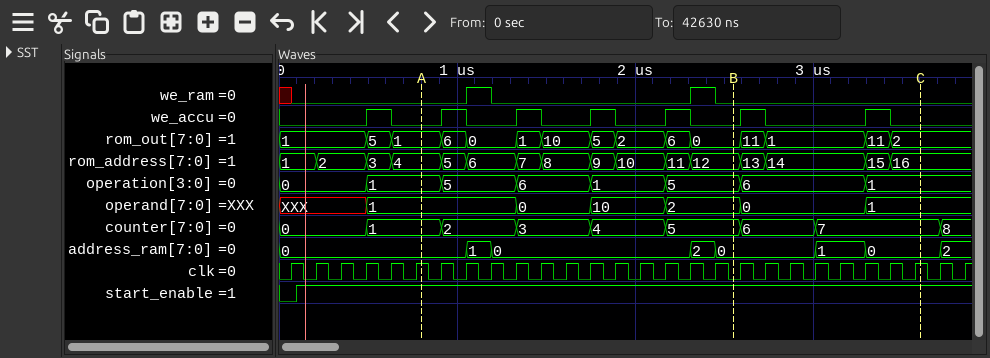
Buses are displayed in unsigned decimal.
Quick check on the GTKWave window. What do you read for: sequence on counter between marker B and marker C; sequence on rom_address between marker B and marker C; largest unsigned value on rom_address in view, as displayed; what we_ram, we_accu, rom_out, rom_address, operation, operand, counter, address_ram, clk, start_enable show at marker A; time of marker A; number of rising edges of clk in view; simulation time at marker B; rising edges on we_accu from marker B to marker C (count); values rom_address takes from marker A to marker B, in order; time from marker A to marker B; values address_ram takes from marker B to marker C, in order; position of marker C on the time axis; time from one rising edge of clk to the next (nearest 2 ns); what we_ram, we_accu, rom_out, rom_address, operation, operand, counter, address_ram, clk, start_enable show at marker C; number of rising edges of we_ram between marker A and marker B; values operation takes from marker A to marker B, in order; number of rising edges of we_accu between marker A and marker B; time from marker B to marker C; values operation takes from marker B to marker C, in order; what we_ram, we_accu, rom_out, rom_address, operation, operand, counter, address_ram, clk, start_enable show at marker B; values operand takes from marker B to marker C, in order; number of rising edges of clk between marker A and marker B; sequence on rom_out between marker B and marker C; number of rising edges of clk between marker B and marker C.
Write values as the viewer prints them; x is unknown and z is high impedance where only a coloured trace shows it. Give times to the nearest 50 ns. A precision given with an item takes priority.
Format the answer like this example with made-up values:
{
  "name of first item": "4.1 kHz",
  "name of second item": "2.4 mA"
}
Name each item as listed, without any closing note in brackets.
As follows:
{
  "sequence on counter between marker B and marker C": "5, 6, 7",
  "sequence on rom_address between marker B and marker C": "12, 13, 14, 15, 16",
  "largest unsigned value on rom_address in view, as displayed": "16",
  "what we_ram, we_accu, rom_out, rom_address, operation, operand, counter, address_ram, clk, start_enable show at marker A": "we_ram=0, we_accu=0, rom_out=1, rom_address=4, operation=1, operand=1, counter=1, address_ram=0, clk=1, start_enable=1",
  "time of marker A": "800 ns",
  "number of rising edges of clk in view": "28",
  "simulation time at marker B": "2550 ns",
  "rising edges on we_accu from marker B to marker C": "2",
  "values rom_address takes from marker A to marker B, in order": "4, 5, 6, 7, 8, 9, 10, 11, 12",
  "time from marker A to marker B": "1750 ns",
  "values address_ram takes from marker B to marker C, in order": "0, 1, 0",
  "position of marker C on the time axis": "3600 ns",
  "time from one rising edge of clk to the next": "140 ns",
  "what we_ram, we_accu, rom_out, rom_address, operation, operand, counter, address_ram, clk, start_enable show at marker C": "we_ram=0, we_accu=0, rom_out=2, rom_address=16, operation=1, operand=1, counter=7, address_ram=0, clk=1, start_enable=1",
  "number of rising edges of we_ram between marker A and marker B": "2",
  "values operation takes from marker A to marker B, in order": "1, 5, 6, 1, 5",
  "number of rising edges of we_accu between marker A and marker B": "4",
  "time from marker B to marker C": "1050 ns",
  "values operation takes from marker B to marker C, in order": "5, 6, 1",
  "what we_ram, we_accu, rom_out, rom_address, operation, operand, counter, address_ram, clk, start_enable show at marker B": "we_ram=0, we_accu=0, rom_out=0, rom_address=12, operation=5, operand=2, counter=5, address_ram=0, clk=0, start_enable=1",
  "values operand takes from marker B to marker C, in order": "2, 0, 1",
  "number of rising edges of clk between marker A and marker B": "12",
  "sequence on rom_out between marker B and marker C": "0, 11, 1, 11, 2",
  "number of rising edges of clk between marker B and marker C": "8"
}
